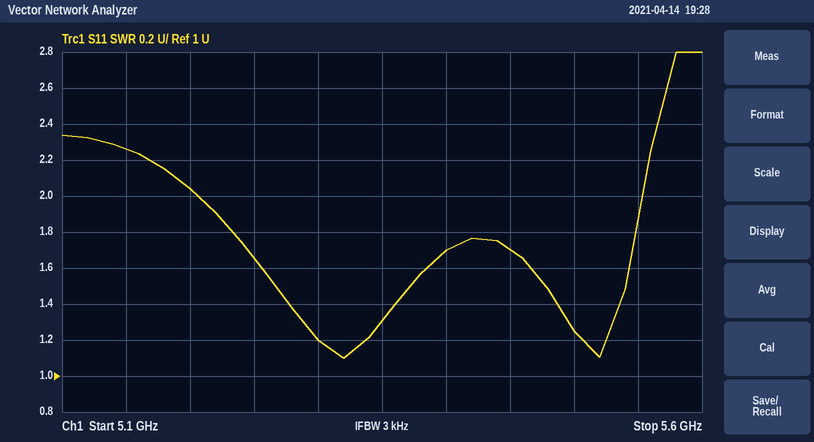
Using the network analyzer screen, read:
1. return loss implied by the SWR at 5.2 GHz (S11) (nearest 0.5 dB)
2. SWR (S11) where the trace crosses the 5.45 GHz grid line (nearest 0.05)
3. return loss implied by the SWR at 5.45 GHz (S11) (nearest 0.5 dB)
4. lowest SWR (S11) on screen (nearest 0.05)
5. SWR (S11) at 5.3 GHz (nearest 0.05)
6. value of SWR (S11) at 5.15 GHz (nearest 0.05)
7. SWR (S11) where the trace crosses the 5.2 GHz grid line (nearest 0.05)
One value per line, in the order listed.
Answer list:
9.5 dB
1.70
11.5 dB
1.10
1.20
2.25
2.05
